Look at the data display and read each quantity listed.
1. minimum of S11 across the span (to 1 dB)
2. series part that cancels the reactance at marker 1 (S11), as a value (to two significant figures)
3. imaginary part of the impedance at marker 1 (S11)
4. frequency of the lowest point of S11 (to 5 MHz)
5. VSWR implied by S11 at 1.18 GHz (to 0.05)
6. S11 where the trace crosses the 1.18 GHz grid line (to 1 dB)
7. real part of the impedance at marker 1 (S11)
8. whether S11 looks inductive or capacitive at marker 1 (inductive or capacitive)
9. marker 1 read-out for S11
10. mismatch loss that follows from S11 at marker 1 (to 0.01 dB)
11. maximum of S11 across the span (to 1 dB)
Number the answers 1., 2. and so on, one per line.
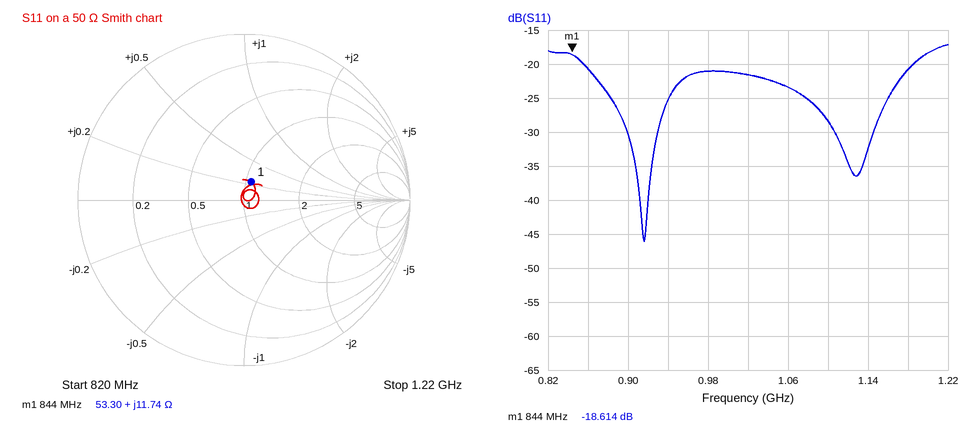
1. -46 dB
2. 16 pF
3. +11.74 Ω
4. 915 MHz
5. 1.20
6. -21 dB
7. 53.30 Ω
8. inductive
9. -18.614 dB
10. 0.06 dB
11. -17 dB
